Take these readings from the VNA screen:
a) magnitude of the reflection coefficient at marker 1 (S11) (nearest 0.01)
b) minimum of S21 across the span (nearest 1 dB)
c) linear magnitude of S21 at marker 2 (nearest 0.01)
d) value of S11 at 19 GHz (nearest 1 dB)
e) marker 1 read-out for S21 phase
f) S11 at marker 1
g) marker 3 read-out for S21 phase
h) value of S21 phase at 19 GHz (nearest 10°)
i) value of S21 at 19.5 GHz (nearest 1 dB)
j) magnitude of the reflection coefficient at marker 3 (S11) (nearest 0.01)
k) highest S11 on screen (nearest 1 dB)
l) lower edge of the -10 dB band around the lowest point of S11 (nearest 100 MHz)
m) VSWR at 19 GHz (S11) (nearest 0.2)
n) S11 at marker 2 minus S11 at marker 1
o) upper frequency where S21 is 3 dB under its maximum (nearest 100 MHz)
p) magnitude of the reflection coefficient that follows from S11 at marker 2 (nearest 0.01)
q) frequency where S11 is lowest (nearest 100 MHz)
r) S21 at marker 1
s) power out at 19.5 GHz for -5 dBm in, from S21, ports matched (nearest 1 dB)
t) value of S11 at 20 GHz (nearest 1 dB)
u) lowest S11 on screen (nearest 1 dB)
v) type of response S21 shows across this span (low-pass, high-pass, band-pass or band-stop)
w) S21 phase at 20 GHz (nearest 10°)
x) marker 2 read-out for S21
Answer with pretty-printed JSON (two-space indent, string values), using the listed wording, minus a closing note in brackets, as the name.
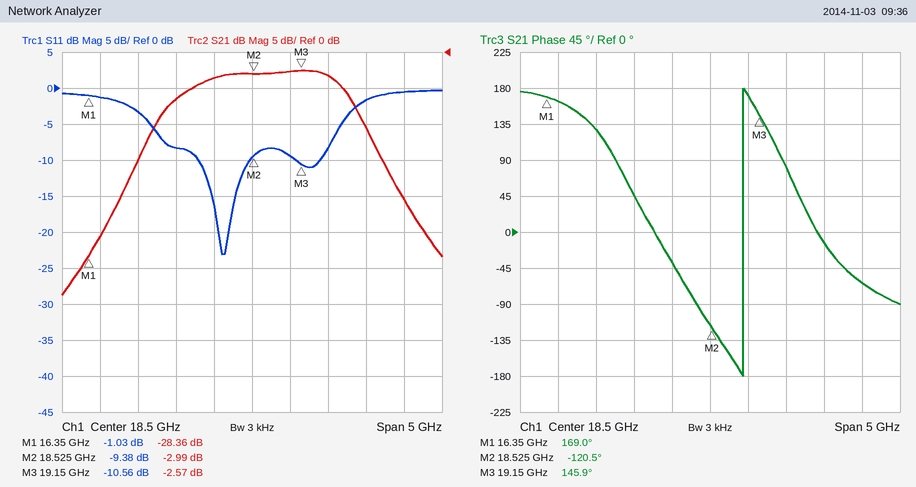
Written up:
{
  "magnitude of the reflection coefficient at marker 1 (S11)": "0.89",
  "minimum of S21 across the span": "-34 dB",
  "linear magnitude of S21 at marker 2": "0.71",
  "value of S11 at 19 GHz": "-9 dB",
  "marker 1 read-out for S21 phase": "169.0°",
  "S11 at marker 1": "-1.03 dB",
  "marker 3 read-out for S21 phase": "145.9°",
  "value of S21 phase at 19 GHz": "170°",
  "value of S21 at 19.5 GHz": "-3 dB",
  "magnitude of the reflection coefficient at marker 3 (S11)": "0.30",
  "highest S11 on screen": "0 dB",
  "lower edge of the -10 dB band around the lowest point of S11": "17.8 GHz",
  "VSWR at 19 GHz (S11)": "2.0",
  "S11 at marker 2 minus S11 at marker 1": "-8.35 dB",
  "upper frequency where S21 is 3 dB under its maximum": "19.7 GHz",
  "magnitude of the reflection coefficient that follows from S11 at marker 2": "0.34",
  "frequency where S11 is lowest": "18.1 GHz",
  "S21 at marker 1": "-28.36 dB",
  "power out at 19.5 GHz for -5 dBm in, from S21, ports matched": "-8 dBm",
  "value of S11 at 20 GHz": "-2 dB",
  "lowest S11 on screen": "-23 dB",
  "type of response S21 shows across this span": "band-pass",
  "S21 phase at 20 GHz": "-10°",
  "marker 2 read-out for S21": "-2.99 dB"
}
